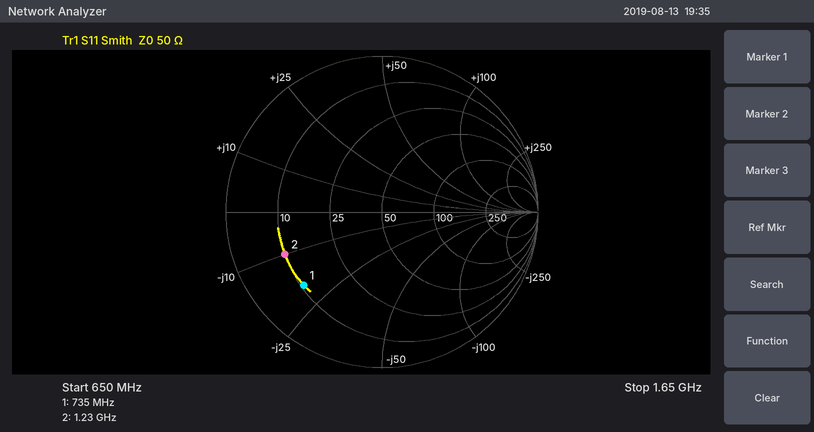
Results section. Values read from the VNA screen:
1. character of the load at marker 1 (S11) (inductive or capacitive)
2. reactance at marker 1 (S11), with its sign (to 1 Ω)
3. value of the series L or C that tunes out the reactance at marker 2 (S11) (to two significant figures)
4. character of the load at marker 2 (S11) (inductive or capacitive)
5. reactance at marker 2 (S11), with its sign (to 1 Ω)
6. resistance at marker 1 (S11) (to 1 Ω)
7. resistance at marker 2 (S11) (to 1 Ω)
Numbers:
capacitive
-19 Ω
1.3 nH
capacitive
-10 Ω
11 Ω
10 Ω
